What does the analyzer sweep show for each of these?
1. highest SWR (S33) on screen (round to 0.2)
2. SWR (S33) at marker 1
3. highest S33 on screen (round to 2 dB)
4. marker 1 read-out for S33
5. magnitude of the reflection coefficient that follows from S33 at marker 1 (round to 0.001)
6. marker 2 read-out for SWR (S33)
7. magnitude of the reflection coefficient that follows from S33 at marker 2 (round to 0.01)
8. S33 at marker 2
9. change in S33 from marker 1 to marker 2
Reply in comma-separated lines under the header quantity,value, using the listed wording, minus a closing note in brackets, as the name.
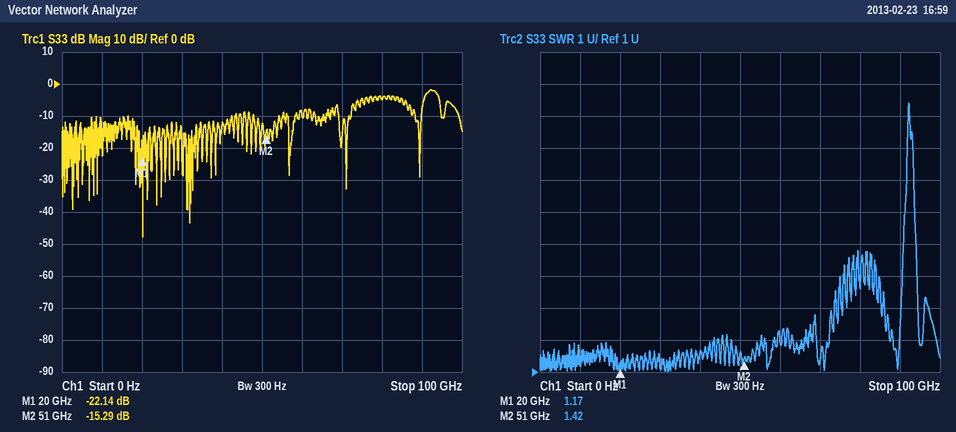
quantity,value
highest SWR (S33) on screen,9.4
SWR (S33) at marker 1,1.17
highest S33 on screen,-2 dB
marker 1 read-out for S33,-22.14 dB
magnitude of the reflection coefficient that follows from S33 at marker 1,0.078
marker 2 read-out for SWR,1.42
magnitude of the reflection coefficient that follows from S33 at marker 2,0.17
S33 at marker 2,-15.29 dB
change in S33 from marker 1 to marker 2,6.85 dB
